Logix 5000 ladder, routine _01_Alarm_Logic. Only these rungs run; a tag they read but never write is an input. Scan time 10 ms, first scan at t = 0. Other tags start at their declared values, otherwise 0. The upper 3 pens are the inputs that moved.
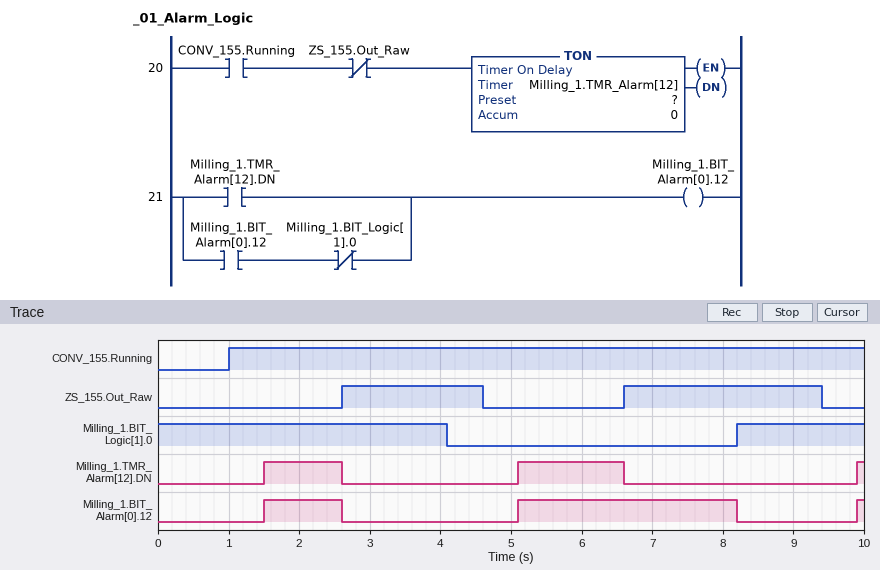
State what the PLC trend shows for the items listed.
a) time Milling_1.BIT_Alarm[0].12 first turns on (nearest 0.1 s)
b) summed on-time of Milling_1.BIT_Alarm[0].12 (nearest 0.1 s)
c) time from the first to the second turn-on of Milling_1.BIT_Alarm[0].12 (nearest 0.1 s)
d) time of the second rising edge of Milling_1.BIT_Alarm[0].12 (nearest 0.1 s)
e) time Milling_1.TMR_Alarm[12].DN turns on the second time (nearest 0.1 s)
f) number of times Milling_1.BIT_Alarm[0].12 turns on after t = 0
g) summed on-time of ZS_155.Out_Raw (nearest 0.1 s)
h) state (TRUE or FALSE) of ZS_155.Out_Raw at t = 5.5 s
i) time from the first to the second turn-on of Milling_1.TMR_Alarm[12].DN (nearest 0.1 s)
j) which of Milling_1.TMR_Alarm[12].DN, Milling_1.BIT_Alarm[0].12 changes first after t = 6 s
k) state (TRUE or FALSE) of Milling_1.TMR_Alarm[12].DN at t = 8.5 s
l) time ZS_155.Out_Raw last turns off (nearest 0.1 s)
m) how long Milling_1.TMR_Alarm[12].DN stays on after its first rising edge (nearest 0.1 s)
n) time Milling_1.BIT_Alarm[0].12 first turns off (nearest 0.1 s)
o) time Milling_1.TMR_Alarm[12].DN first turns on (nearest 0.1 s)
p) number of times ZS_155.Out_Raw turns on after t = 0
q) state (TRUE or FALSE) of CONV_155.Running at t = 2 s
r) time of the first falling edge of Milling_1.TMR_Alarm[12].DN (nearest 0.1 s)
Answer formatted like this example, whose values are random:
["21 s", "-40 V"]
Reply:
["1.5 s", "4.3 s", "3.6 s", "5.1 s", "5.1 s", "3", "4.8 s", "FALSE", "3.6 s", "Milling_1.TMR_Alarm[12].DN", "FALSE", "9.4 s", "1.1 s", "2.6 s", "1.5 s", "2", "TRUE", "2.6 s"]
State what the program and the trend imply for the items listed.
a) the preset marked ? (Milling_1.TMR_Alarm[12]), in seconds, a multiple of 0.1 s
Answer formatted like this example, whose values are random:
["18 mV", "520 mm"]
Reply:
["0.5 s"]
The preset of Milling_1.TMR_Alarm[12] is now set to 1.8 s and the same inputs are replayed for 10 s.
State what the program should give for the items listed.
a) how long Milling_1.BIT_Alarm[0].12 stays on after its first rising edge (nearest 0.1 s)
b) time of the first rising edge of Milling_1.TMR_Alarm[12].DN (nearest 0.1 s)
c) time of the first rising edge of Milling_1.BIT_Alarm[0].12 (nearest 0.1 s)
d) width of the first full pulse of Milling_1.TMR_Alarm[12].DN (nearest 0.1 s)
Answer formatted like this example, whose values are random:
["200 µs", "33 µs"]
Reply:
["1.8 s", "6.4 s", "6.4 s", "0.2 s"]
